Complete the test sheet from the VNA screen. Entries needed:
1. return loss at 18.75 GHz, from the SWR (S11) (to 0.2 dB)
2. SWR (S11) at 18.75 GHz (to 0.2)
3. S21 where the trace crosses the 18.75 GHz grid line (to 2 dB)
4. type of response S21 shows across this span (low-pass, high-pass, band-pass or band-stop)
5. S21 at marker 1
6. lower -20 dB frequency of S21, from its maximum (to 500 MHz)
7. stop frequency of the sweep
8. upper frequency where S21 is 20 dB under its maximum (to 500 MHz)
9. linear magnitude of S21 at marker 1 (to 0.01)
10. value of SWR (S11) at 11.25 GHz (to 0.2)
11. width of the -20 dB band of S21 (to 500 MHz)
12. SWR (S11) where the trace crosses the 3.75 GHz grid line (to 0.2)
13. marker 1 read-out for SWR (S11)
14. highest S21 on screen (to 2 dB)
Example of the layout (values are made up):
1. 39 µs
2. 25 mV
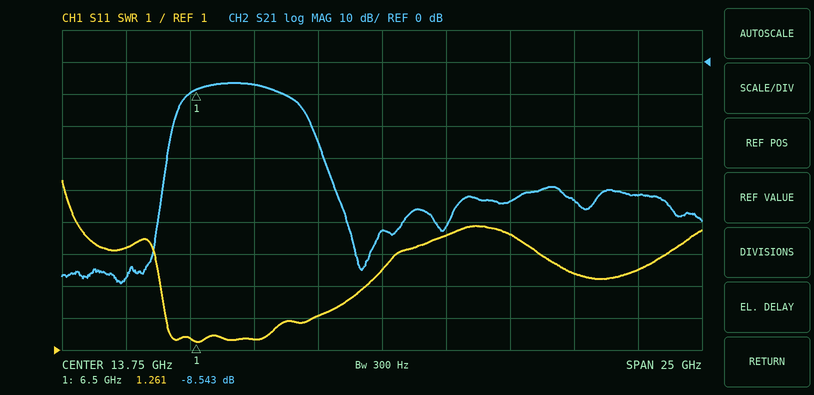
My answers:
1. 3.8 dB
2. 4.6
3. -44 dB
4. band-pass
5. -8.543 dB
6. 5.5 GHz
7. 26.25 GHz
8. 11.5 GHz
9. 0.37
10. 2.0
11. 6.0 GHz
12. 4.2
13. 1.261
14. -6 dB
